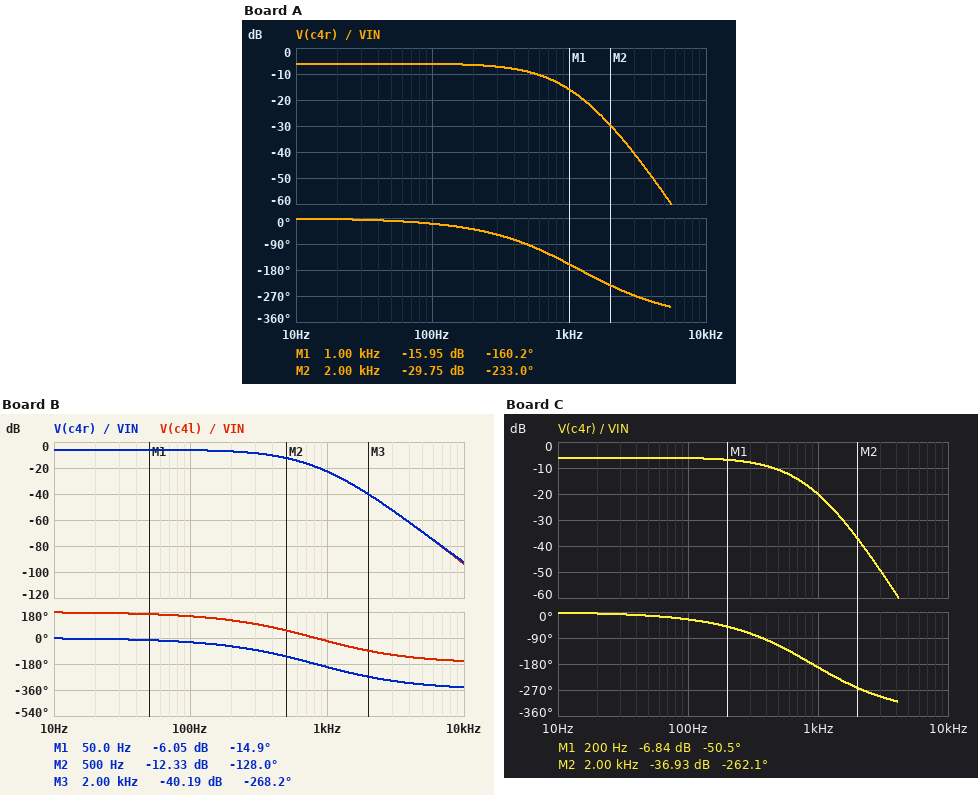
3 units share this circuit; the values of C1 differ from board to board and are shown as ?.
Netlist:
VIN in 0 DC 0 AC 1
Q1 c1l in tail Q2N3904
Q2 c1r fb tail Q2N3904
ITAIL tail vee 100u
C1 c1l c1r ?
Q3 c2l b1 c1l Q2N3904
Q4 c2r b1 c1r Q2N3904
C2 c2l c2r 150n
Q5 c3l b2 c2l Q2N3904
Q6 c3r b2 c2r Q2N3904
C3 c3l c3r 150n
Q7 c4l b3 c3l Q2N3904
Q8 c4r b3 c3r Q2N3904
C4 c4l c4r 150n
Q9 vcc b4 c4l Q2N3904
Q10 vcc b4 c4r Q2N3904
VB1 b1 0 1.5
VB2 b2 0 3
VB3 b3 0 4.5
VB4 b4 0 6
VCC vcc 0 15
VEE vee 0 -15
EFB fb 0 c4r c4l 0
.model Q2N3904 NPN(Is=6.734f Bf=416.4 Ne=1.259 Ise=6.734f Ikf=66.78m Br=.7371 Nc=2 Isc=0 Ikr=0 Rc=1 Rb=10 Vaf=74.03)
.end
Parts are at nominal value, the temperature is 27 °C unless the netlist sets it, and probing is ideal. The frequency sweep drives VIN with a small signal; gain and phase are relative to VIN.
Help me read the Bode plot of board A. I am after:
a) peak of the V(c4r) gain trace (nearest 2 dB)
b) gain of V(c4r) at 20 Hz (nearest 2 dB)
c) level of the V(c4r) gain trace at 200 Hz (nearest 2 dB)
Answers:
-6 dB
-6 dB
-6 dB
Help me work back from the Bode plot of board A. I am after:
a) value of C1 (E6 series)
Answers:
68 nF
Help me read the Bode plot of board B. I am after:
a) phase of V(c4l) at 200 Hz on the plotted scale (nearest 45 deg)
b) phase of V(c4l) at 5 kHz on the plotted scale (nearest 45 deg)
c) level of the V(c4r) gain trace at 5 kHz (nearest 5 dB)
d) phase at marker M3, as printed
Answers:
135 deg
-135 deg
-70 dB
-268.2 deg
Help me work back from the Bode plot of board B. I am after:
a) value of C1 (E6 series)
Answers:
330 nF
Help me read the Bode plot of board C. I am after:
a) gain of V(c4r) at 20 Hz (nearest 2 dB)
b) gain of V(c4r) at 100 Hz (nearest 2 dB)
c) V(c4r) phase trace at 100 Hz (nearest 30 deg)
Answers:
-6 dB
-6 dB
-30 deg
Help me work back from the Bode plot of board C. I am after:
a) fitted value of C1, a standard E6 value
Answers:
220 nF
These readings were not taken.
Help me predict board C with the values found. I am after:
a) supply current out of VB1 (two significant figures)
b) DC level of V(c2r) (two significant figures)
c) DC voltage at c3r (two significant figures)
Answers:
1.1 µA
2.4 V
3.9 V
